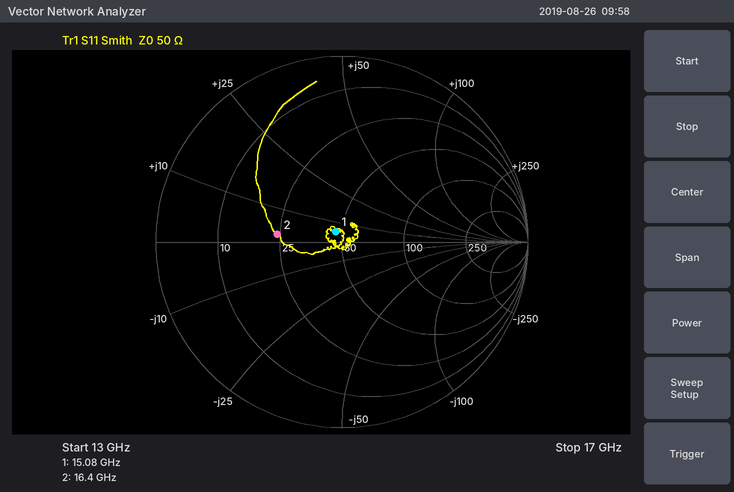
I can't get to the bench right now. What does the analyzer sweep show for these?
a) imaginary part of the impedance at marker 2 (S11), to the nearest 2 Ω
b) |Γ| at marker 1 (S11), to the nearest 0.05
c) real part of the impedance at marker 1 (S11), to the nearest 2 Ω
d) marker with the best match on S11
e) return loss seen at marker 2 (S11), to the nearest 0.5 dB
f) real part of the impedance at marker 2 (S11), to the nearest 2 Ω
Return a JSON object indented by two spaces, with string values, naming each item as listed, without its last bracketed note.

{
  "imaginary part of the impedance at marker 2 (S11), to the nearest 2 Ω": "+2 Ω",
  "|Γ| at marker 1 (S11), to the nearest 0.05": "0.05",
  "real part of the impedance at marker 1 (S11), to the nearest 2 Ω": "46 Ω",
  "marker with the best match on S11": "marker 1",
  "return loss seen at marker 2 (S11), to the nearest 0.5 dB": "9.0 dB",
  "real part of the impedance at marker 2 (S11), to the nearest 2 Ω": "24 Ω"
}
